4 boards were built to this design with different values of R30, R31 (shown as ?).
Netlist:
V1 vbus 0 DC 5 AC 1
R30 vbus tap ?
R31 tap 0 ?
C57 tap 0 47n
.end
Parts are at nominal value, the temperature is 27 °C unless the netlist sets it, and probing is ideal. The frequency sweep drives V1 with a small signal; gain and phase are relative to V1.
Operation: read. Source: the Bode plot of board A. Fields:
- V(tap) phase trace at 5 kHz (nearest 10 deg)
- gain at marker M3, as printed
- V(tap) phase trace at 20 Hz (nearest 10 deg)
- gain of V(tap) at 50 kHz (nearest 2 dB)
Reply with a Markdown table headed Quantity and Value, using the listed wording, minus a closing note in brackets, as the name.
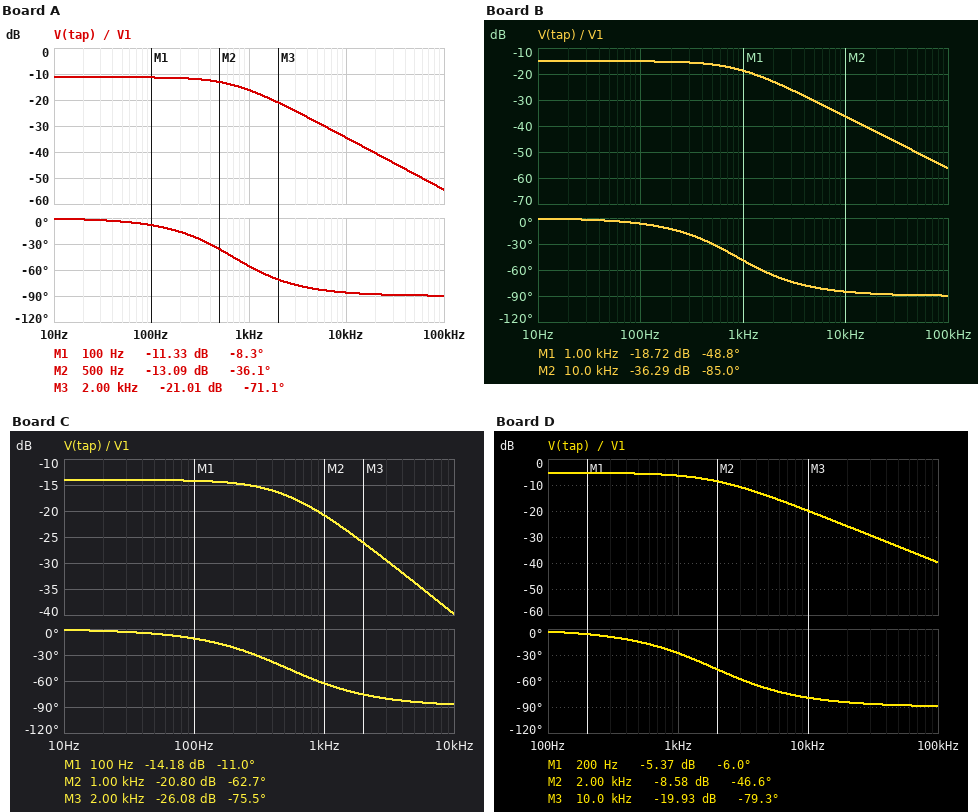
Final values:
| Quantity | Value |
|---|---|
| V(tap) phase trace at 5 kHz | -80 deg |
| gain at marker M3, as printed | -21.01 dB |
| V(tap) phase trace at 20 Hz | 0 deg |
| gain of V(tap) at 50 kHz | -48 dB |
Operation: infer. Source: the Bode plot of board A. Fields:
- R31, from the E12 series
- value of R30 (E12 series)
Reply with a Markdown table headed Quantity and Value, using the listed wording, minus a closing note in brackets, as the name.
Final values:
| Quantity | Value |
|---|---|
| R31, from the E12 series | 6.8 kΩ |
| value of R30 | 18 kΩ |
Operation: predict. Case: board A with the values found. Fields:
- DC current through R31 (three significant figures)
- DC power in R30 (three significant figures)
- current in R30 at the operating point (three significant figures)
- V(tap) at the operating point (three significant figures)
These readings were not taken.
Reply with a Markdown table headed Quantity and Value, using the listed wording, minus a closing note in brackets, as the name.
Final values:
| Quantity | Value |
|---|---|
| DC current through R31 | 202 µA |
| DC power in R30 | 732 µW |
| current in R30 at the operating point | 202 µA |
| V(tap) at the operating point | 1.37 V |
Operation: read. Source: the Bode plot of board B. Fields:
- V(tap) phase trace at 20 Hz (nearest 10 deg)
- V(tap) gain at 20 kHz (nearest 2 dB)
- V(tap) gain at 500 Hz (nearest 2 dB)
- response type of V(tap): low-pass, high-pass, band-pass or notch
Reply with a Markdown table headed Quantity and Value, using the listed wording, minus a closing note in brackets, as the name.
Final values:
| Quantity | Value |
|---|---|
| V(tap) phase trace at 20 Hz | 0 deg |
| V(tap) gain at 20 kHz | -42 dB |
| V(tap) gain at 500 Hz | -16 dB |
| response type of V(tap): low-pass, high-pass, band-pass or notch | low-pass |
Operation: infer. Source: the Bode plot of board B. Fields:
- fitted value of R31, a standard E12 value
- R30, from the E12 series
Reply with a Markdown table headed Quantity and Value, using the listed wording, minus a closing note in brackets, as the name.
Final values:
| Quantity | Value |
|---|---|
| fitted value of R31, a standard E12 value | 4.7 kΩ |
| R30, from the E12 series | 22 kΩ |
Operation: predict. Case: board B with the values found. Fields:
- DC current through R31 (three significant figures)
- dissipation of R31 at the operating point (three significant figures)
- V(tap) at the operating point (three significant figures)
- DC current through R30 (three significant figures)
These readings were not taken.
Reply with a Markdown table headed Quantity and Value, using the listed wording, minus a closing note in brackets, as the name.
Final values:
| Quantity | Value |
|---|---|
| DC current through R31 | 187 µA |
| dissipation of R31 at the operating point | 165 µW |
| V(tap) at the operating point | 880 mV |
| DC current through R30 | 187 µA |
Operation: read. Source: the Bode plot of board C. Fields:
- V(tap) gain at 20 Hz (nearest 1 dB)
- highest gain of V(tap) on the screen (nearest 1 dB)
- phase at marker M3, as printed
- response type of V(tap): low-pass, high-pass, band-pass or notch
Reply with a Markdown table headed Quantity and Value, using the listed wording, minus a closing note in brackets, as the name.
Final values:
| Quantity | Value |
|---|---|
| V(tap) gain at 20 Hz | -14 dB |
| highest gain of V(tap) on the screen | -14 dB |
| phase at marker M3, as printed | -75.5 deg |
| response type of V(tap): low-pass, high-pass, band-pass or notch | low-pass |
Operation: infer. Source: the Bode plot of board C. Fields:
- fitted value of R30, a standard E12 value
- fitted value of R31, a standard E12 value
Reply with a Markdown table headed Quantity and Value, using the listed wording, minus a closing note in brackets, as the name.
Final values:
| Quantity | Value |
|---|---|
| fitted value of R30, a standard E12 value | 33 kΩ |
| fitted value of R31, a standard E12 value | 8.2 kΩ |
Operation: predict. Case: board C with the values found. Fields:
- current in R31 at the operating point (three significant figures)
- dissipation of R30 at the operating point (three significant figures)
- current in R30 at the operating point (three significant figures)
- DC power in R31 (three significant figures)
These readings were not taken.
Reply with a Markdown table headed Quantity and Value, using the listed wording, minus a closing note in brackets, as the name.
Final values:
| Quantity | Value |
|---|---|
| current in R31 at the operating point | 121 µA |
| dissipation of R30 at the operating point | 486 µW |
| current in R30 at the operating point | 121 µA |
| DC power in R31 | 121 µW |
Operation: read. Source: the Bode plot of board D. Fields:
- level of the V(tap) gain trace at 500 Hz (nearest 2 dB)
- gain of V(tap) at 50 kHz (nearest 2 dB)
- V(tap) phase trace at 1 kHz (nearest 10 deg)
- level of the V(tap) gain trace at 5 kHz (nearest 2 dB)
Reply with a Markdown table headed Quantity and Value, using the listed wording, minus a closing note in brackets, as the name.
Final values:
| Quantity | Value |
|---|---|
| level of the V(tap) gain trace at 500 Hz | -6 dB |
| gain of V(tap) at 50 kHz | -34 dB |
| V(tap) phase trace at 1 kHz | -30 deg |
| level of the V(tap) gain trace at 5 kHz | -14 dB |
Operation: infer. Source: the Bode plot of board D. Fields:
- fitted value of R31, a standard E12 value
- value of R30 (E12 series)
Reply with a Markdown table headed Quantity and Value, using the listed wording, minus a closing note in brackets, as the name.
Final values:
| Quantity | Value |
|---|---|
| fitted value of R31, a standard E12 value | 3.9 kΩ |
| value of R30 | 3.3 kΩ |
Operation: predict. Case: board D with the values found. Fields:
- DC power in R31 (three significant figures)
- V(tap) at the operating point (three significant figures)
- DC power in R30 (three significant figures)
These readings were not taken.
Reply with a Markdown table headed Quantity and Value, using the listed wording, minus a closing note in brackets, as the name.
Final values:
| Quantity | Value |
|---|---|
| DC power in R31 | 1.88 mW |
| V(tap) at the operating point | 2.71 V |
| DC power in R30 | 1.59 mW |
